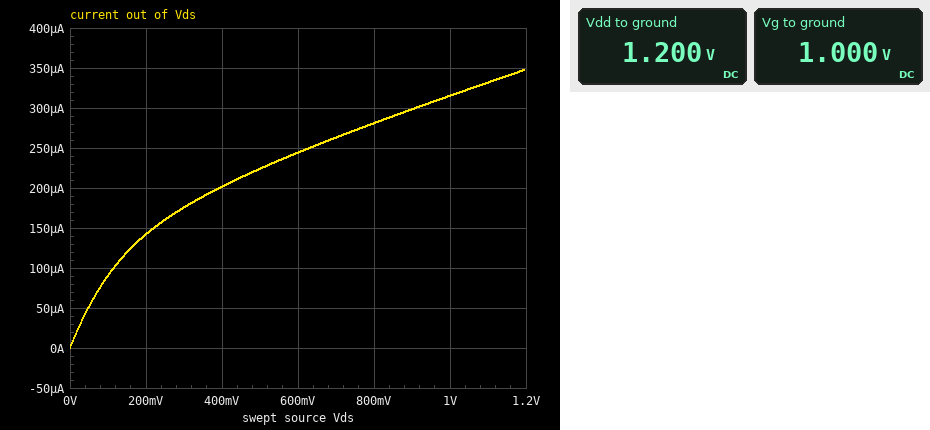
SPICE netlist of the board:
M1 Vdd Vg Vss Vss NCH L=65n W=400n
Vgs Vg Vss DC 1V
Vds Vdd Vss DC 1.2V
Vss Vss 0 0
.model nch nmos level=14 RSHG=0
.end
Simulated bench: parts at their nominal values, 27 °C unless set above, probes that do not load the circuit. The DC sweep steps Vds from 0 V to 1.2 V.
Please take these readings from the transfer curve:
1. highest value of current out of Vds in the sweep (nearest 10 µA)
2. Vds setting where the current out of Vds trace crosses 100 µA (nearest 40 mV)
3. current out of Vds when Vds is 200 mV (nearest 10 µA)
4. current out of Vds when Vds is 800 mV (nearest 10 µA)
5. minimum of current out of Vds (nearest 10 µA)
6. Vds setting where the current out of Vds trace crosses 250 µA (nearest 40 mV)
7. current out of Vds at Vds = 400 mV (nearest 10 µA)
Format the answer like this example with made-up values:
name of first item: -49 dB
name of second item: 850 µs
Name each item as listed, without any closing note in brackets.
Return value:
highest value of current out of Vds in the sweep: 350 µA
Vds setting where the current out of Vds trace crosses 100 µA: 120 mV
current out of Vds when Vds is 200 mV: 140 µA
current out of Vds when Vds is 800 mV: 280 µA
minimum of current out of Vds: 0 A
Vds setting where the current out of Vds trace crosses 250 µA: 640 mV
current out of Vds at Vds = 400 mV: 200 µA
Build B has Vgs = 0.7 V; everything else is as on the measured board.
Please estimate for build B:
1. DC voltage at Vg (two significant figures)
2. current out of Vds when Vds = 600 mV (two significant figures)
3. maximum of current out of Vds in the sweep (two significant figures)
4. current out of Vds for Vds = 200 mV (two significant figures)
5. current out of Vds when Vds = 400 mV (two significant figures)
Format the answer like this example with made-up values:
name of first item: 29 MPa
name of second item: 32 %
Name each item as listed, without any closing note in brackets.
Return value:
DC voltage at Vg: 700 mV
current out of Vds when Vds = 600 mV: 150 µA
maximum of current out of Vds in the sweep: 230 µA
current out of Vds for Vds = 200 mV: 81 µA
current out of Vds when Vds = 400 mV: 120 µA
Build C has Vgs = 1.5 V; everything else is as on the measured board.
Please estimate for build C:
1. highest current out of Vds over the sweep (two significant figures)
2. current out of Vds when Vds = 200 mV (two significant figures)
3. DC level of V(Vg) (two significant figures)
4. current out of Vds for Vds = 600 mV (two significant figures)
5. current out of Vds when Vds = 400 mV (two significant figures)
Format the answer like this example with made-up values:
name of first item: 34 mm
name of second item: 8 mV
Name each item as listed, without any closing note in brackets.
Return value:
highest current out of Vds over the sweep: 540 µA
current out of Vds when Vds = 200 mV: 230 µA
DC level of V(Vg): 1.5 V
current out of Vds for Vds = 600 mV: 400 µA
current out of Vds when Vds = 400 mV: 340 µA
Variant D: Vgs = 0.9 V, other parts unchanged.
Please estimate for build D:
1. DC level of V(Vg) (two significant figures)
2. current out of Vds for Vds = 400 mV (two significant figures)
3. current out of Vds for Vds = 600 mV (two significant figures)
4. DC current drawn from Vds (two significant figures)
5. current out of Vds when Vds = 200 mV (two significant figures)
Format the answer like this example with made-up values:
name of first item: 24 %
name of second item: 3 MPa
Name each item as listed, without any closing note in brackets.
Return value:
DC level of V(Vg): 900 mV
current out of Vds for Vds = 400 mV: 170 µA
current out of Vds for Vds = 600 mV: 210 µA
DC current drawn from Vds: 310 µA
current out of Vds when Vds = 200 mV: 120 µA
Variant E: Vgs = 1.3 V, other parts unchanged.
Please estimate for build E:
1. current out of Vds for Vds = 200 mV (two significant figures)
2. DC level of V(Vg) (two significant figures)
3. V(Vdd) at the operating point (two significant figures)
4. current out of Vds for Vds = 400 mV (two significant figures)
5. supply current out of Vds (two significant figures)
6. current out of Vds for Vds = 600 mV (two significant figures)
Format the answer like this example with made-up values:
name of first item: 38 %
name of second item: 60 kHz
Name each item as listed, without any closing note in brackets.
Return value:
current out of Vds for Vds = 200 mV: 200 µA
DC level of V(Vg): 1.3 V
V(Vdd) at the operating point: 1.2 V
current out of Vds for Vds = 400 mV: 280 µA
supply current out of Vds: 460 µA
current out of Vds for Vds = 600 mV: 340 µA
